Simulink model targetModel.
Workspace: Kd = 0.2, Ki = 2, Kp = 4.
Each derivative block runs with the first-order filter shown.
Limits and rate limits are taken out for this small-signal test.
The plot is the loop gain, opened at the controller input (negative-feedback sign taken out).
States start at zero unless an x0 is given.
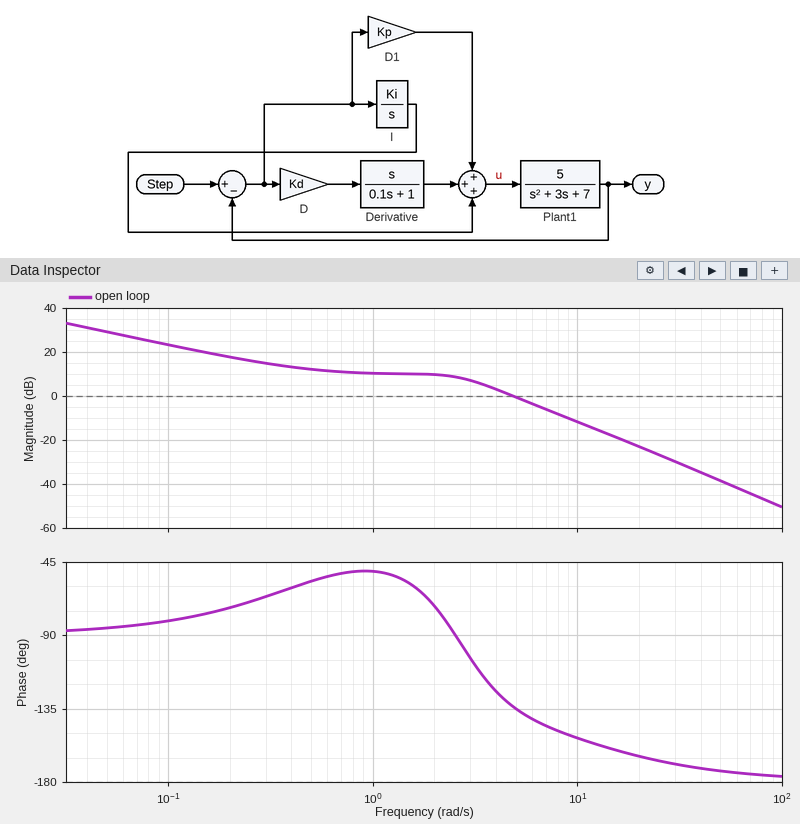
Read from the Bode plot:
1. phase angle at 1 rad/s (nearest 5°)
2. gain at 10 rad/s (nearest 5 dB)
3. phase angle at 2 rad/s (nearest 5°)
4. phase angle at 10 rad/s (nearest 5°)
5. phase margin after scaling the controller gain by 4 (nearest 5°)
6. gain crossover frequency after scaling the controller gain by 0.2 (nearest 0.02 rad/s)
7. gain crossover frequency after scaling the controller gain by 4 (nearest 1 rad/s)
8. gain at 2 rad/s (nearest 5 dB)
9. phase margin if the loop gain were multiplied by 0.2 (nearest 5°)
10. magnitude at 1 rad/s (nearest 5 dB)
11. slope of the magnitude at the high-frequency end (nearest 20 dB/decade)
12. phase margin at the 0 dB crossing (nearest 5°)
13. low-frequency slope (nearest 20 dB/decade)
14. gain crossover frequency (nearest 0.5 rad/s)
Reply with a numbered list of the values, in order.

1. -50°
2. -10 dB
3. -70°
4. -155°
5. 25°
6. 0.34 rad/s
7. 10 rad/s
8. 10 dB
9. 115°
10. 10 dB
11. -40 dB/decade
12. 45°
13. -20 dB/decade
14. 5.0 rad/s
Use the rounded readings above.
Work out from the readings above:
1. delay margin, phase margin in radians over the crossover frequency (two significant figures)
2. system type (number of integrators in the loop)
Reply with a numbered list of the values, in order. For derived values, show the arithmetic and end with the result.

1. 45 × π / 180 / 5 = 0.16 s
2. 1
